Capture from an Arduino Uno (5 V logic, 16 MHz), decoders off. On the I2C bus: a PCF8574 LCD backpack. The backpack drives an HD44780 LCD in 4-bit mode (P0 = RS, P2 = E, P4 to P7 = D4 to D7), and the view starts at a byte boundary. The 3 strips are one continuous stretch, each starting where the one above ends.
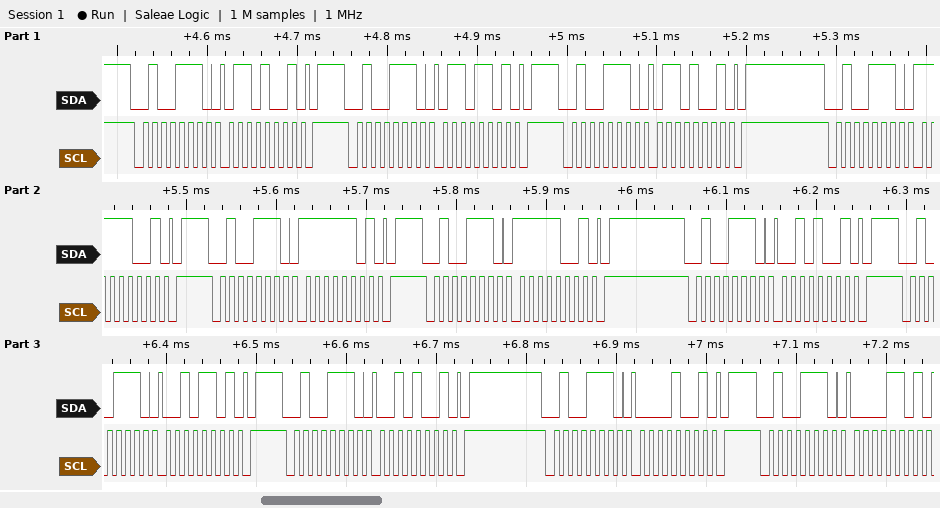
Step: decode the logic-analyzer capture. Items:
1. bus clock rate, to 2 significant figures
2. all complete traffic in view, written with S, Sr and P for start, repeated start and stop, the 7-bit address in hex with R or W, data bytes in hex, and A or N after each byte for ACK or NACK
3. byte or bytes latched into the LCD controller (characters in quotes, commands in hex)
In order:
100 kHz
S 27W A 69 A P S 27W A 6D A P S 27W A 69 A P S 27W A F9 A P S 27W A FD A P S 27W A F9 A P S 27W A 29 A P S 27W A 2D A P S 27W A 29 A P S 27W A 09 A P S 27W A 0D A
'o'
